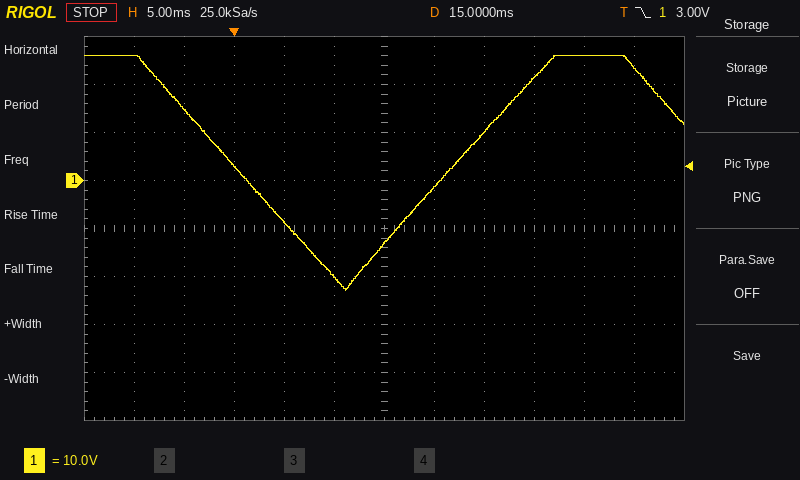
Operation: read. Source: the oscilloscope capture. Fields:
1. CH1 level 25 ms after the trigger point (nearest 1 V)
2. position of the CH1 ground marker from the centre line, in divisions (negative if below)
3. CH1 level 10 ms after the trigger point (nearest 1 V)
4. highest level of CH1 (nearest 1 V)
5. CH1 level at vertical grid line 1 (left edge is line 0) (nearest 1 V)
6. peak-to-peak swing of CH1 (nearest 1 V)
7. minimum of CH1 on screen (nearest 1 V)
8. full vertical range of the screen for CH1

10 V
+1.0 div
-20 V
26 V
26 V
49 V
-23 V
80 V
